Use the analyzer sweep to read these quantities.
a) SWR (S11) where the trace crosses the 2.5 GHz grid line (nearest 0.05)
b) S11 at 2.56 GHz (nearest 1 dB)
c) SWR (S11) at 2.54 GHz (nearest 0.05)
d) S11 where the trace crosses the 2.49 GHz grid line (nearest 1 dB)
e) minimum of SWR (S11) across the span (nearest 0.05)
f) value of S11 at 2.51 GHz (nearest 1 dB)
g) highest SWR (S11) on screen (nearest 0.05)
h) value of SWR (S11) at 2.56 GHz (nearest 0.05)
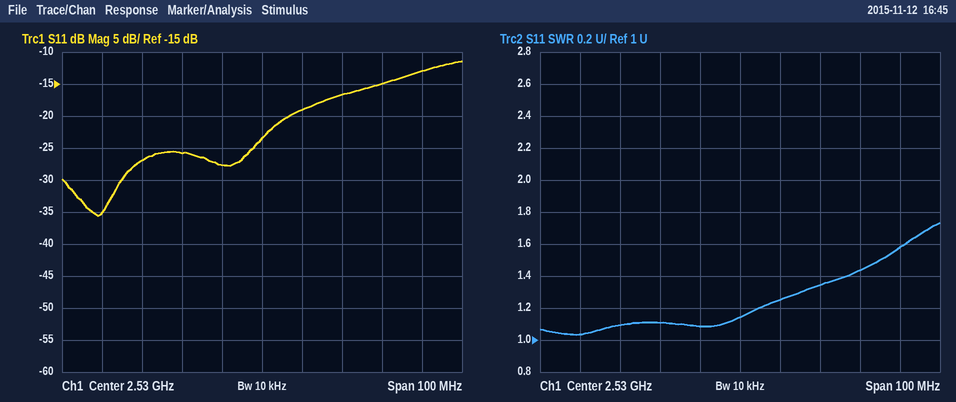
1.10
-15 dB
1.25
-35 dB
1.05
-26 dB
1.75
1.45
